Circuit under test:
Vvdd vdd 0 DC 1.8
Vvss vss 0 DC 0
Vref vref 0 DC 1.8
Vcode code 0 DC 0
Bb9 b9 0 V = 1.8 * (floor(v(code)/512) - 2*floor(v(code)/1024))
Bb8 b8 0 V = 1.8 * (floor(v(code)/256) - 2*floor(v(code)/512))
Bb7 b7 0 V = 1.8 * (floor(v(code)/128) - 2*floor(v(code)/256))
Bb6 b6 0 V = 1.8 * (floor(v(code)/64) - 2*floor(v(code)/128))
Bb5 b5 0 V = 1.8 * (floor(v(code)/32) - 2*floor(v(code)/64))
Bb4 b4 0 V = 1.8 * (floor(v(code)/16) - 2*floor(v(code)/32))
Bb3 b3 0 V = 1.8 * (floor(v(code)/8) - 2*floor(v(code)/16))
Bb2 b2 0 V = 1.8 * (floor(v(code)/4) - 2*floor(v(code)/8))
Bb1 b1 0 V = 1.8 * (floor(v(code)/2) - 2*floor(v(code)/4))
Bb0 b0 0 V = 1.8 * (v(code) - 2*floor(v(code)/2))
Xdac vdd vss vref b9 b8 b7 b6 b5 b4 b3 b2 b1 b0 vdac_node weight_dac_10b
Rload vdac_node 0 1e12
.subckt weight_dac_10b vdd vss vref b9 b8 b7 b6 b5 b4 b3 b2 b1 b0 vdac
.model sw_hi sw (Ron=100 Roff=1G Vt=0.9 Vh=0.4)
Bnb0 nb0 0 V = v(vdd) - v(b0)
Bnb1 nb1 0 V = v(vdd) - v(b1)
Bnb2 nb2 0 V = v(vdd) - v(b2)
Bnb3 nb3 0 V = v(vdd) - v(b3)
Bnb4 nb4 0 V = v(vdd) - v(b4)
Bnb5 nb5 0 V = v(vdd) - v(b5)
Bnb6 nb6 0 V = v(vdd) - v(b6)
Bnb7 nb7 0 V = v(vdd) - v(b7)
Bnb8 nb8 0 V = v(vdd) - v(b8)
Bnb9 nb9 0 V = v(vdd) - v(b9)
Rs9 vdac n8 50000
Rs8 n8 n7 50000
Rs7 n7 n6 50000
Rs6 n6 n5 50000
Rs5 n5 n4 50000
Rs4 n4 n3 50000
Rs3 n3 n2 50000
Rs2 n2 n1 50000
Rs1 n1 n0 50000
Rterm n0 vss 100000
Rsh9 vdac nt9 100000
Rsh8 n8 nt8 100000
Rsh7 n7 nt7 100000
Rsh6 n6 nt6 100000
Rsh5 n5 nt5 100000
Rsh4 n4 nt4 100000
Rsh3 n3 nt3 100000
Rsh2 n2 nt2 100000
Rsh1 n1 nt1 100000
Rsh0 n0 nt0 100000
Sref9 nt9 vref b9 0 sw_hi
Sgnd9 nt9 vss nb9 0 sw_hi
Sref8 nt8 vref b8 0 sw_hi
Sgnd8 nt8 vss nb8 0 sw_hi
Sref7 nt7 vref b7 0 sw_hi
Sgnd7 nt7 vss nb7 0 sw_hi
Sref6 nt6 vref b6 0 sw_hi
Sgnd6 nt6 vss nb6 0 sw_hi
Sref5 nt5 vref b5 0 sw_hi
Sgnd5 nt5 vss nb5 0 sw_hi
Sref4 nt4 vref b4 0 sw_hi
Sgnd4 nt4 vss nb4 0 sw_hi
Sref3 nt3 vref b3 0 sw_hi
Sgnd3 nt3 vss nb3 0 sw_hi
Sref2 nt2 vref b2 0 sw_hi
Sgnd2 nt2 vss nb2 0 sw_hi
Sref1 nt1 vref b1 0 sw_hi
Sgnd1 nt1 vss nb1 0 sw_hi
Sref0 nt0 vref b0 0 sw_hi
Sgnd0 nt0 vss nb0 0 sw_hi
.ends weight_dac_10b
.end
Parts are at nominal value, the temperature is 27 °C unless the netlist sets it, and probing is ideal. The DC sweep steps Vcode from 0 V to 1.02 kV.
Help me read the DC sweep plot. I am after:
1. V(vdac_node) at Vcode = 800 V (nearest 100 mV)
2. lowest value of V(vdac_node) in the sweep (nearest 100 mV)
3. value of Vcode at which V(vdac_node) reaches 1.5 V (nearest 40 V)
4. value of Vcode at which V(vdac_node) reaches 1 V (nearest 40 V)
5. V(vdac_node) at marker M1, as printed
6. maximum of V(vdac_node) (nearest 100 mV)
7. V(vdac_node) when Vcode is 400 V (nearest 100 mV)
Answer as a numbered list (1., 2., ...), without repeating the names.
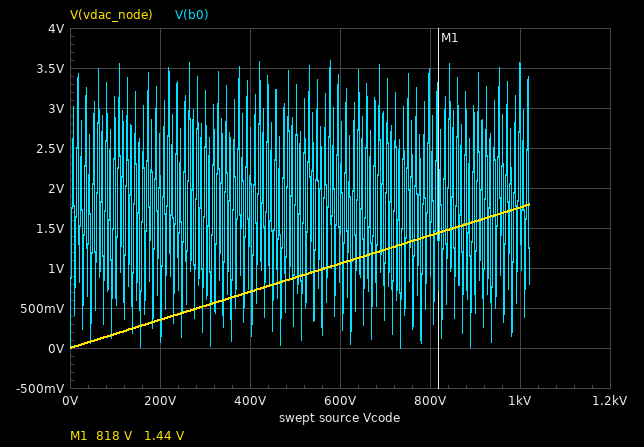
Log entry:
1. 1.4 V
2. 0 V
3. 840 V
4. 560 V
5. 1.44 V
6. 1.8 V
7. 700 mV
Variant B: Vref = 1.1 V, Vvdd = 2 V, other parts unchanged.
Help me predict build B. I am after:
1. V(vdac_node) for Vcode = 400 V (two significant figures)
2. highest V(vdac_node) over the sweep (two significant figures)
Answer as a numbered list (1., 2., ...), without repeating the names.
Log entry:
1. 430 mV
2. 1.1 V
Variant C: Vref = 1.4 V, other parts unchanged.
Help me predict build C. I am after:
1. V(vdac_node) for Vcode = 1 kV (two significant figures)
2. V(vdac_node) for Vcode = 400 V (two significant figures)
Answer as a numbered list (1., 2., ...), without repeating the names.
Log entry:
1. 1.4 V
2. 550 mV
